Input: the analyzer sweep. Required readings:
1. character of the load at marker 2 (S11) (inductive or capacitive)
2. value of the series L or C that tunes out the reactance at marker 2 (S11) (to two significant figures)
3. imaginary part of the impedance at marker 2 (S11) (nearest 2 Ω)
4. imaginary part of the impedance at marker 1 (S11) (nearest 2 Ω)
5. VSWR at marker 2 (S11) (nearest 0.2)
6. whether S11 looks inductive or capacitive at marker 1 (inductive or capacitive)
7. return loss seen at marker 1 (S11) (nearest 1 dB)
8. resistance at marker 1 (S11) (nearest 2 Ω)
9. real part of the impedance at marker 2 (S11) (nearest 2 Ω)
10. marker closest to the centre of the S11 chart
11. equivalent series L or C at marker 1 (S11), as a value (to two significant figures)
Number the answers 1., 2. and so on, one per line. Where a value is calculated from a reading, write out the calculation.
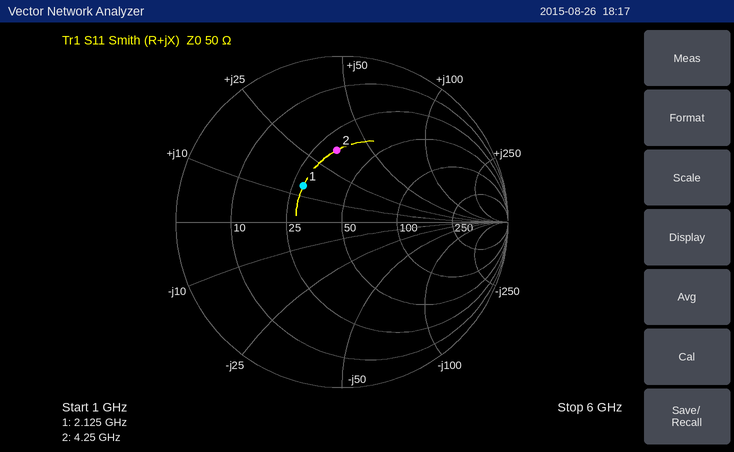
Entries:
1. inductive
2. C = 1/(2π × 4.25 GHz × 34 Ω) ≈ 1.1 pF
3. +34 Ω
4. +14 Ω
5. 2.6
6. inductive
7. 10 dB
8. 28 Ω
9. 32 Ω
10. marker 1
11. L = 14 Ω/(2π × 2.125 GHz) ≈ 1.0 nH
